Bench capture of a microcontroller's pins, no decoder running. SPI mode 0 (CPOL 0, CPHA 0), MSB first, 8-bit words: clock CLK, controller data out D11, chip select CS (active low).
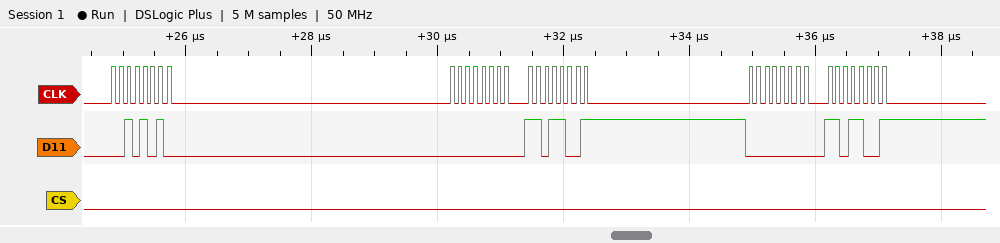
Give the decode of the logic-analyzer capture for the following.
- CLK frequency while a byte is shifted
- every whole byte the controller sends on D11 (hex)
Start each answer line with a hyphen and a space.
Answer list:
- 8 MHz
- 2A 00 D9 00 D9
